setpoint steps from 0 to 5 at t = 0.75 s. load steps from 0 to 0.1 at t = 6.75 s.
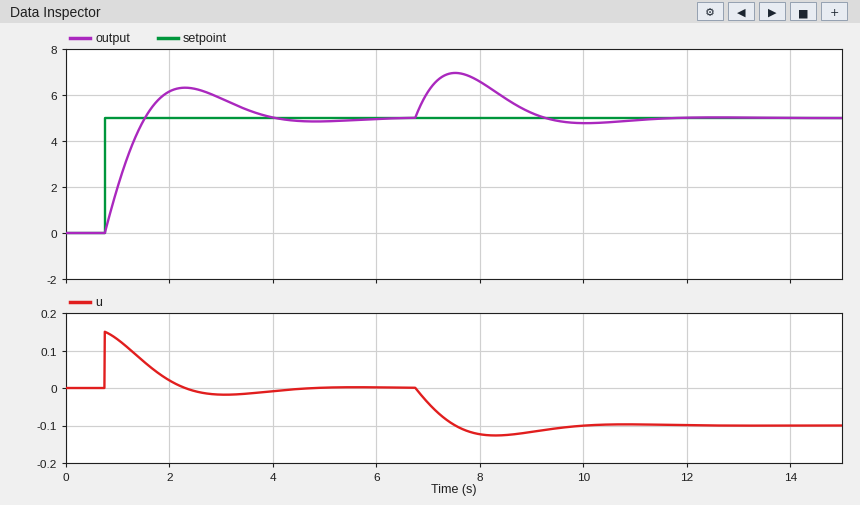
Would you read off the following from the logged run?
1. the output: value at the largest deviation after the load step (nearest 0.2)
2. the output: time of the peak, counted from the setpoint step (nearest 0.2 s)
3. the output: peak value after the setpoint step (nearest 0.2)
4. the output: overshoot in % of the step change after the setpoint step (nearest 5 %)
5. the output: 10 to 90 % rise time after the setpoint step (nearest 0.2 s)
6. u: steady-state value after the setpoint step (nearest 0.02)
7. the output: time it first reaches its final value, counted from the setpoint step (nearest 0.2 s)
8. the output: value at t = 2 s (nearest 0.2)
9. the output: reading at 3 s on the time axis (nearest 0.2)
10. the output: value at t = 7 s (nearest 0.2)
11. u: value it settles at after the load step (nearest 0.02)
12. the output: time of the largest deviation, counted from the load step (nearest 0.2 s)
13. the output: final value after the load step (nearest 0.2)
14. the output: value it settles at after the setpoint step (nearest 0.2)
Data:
7.0
1.6 s
6.4
25 %
0.6 s
0.00
0.8 s
6.2
5.8
6.2
-0.10
0.8 s
5.0
5.0
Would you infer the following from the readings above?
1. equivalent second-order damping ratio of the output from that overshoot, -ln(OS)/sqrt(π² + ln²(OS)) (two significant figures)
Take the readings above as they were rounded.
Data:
0.40
